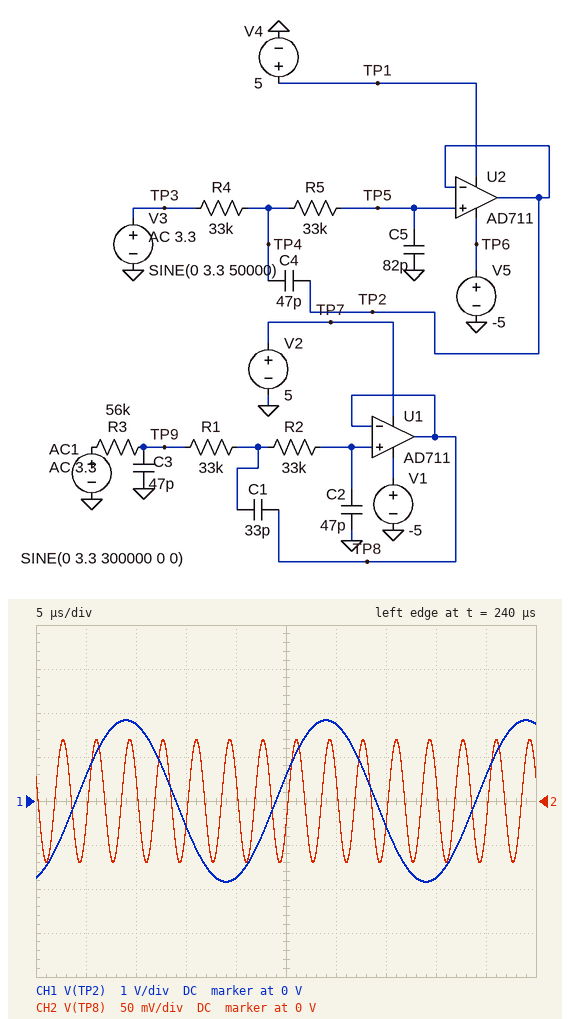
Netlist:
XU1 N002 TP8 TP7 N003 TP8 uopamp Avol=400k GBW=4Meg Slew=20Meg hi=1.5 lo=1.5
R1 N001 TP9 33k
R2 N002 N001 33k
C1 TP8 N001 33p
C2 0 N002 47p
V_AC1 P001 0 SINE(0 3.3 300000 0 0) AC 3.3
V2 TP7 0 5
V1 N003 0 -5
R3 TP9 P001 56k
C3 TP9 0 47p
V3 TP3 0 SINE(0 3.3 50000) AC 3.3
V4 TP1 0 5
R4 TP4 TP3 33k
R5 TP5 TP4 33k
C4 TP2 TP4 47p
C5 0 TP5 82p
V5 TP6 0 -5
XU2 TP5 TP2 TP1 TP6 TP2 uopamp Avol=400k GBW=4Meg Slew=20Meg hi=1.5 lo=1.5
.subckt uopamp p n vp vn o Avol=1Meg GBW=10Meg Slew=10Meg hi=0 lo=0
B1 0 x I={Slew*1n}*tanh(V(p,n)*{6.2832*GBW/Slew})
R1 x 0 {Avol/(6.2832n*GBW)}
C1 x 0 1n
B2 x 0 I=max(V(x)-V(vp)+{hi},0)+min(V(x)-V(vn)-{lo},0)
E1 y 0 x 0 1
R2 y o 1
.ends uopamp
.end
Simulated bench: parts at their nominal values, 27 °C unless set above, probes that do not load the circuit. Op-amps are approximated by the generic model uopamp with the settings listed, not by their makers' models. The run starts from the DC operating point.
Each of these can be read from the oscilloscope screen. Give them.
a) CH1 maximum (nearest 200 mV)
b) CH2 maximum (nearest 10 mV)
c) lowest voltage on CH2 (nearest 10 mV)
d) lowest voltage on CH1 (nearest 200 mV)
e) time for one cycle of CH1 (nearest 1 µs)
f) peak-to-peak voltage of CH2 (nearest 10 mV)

1.8 V
70 mV
-70 mV
-1.8 V
20 µs
140 mV
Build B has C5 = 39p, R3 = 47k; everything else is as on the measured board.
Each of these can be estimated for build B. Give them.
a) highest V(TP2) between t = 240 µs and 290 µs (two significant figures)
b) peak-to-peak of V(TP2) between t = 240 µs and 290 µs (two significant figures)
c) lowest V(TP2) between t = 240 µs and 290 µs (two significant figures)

2.9 V
5.8 V
-2.9 V
